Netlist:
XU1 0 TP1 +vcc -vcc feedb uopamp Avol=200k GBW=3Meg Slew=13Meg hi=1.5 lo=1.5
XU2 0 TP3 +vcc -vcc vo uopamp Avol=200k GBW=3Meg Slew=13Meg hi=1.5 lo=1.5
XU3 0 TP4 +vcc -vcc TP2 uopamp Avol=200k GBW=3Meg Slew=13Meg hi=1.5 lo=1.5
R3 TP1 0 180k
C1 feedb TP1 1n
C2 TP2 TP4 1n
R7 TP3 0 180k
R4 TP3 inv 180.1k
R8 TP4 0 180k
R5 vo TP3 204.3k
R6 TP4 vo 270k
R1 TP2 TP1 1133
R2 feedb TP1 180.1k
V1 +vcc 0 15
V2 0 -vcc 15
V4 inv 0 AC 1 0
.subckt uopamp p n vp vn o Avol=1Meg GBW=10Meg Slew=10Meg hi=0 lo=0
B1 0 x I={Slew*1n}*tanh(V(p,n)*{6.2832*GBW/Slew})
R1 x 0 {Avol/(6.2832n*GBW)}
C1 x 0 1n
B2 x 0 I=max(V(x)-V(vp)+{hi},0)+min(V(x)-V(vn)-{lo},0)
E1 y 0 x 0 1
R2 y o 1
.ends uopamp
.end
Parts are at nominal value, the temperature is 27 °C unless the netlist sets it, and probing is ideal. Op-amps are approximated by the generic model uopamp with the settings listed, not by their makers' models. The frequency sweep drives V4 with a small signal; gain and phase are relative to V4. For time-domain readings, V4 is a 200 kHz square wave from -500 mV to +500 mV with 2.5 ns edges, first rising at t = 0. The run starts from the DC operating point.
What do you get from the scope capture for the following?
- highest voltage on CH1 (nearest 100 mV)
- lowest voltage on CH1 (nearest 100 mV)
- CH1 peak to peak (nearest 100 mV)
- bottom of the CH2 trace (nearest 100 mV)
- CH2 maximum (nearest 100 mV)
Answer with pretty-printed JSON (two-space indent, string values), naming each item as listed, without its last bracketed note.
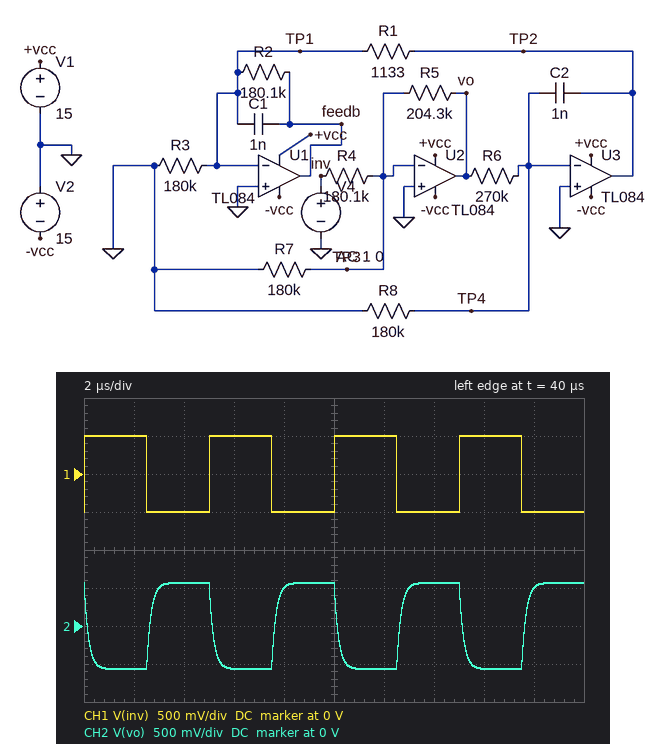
{
  "highest voltage on CH1": "500 mV",
  "lowest voltage on CH1": "-500 mV",
  "CH1 peak to peak": "1.0 V",
  "bottom of the CH2 trace": "-600 mV",
  "CH2 maximum": "600 mV"
}
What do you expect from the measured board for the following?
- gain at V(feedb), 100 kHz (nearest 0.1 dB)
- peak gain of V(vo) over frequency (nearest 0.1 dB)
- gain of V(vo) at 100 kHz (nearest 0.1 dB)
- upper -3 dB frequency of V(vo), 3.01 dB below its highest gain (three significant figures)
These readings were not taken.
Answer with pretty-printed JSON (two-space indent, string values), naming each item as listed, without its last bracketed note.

{
  "gain at V(feedb), 100 kHz": "-41.0 dB",
  "peak gain of V(vo) over frequency": "1.1 dB",
  "gain of V(vo) at 100 kHz": "1.0 dB",
  "upper -3 dB frequency of V(vo), 3.01 dB below its highest gain": "918 kHz"
}
